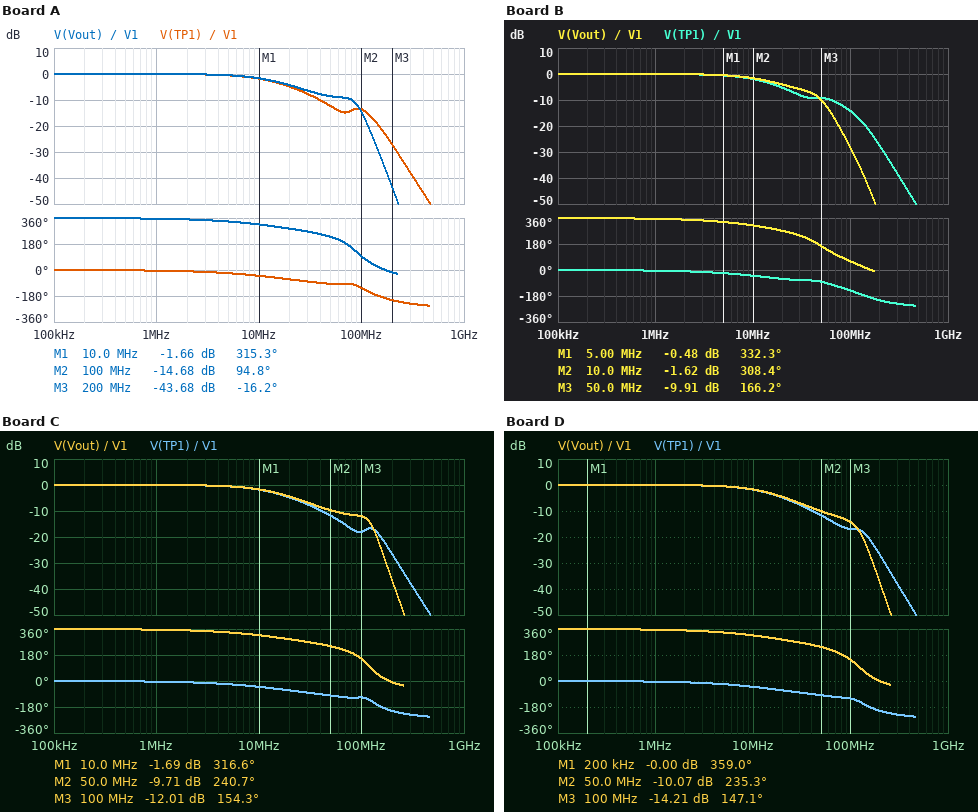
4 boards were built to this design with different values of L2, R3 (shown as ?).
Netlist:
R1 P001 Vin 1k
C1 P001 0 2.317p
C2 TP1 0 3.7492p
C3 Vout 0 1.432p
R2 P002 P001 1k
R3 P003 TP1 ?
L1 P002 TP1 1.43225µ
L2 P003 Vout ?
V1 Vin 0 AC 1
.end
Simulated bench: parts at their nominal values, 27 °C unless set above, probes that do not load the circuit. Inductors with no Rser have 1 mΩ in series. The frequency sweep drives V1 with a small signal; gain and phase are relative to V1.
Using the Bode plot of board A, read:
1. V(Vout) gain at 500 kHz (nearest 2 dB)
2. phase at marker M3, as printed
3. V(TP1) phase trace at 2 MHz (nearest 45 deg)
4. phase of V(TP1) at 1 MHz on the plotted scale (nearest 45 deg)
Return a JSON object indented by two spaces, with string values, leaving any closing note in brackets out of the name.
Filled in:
{
  "V(Vout) gain at 500 kHz": "0 dB",
  "phase at marker M3, as printed": "-16.2 deg",
  "V(TP1) phase trace at 2 MHz": "0 deg",
  "phase of V(TP1) at 1 MHz on the plotted scale": "0 deg"
}
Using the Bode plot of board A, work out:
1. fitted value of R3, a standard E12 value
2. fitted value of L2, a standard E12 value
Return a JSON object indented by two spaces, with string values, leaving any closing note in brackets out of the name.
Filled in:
{
  "fitted value of R3, a standard E12 value": "820 Ω",
  "fitted value of L2, a standard E12 value": "3.3 µH"
}
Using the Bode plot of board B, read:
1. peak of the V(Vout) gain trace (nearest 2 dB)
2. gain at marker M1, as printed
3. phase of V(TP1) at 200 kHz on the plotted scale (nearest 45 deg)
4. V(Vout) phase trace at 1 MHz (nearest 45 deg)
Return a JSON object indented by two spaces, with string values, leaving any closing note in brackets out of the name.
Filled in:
{
  "peak of the V(Vout) gain trace": "0 dB",
  "gain at marker M1, as printed": "-0.48 dB",
  "phase of V(TP1) at 200 kHz on the plotted scale": "0 deg",
  "V(Vout) phase trace at 1 MHz": "360 deg"
}
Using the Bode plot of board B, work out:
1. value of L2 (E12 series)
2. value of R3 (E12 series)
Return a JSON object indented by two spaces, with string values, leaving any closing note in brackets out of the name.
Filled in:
{
  "value of L2": "10 µH",
  "value of R3": "2.2 kΩ"
}
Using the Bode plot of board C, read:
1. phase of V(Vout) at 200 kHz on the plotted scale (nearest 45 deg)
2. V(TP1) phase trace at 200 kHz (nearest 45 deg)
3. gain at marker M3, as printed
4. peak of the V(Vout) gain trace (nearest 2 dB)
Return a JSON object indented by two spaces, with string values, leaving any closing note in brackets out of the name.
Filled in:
{
  "phase of V(Vout) at 200 kHz on the plotted scale": "360 deg",
  "V(TP1) phase trace at 200 kHz": "0 deg",
  "gain at marker M3, as printed": "-12.01 dB",
  "peak of the V(Vout) gain trace": "0 dB"
}
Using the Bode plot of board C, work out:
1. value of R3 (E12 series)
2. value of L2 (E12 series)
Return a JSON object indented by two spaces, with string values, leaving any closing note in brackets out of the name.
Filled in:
{
  "value of R3": "560 Ω",
  "value of L2": "1.8 µH"
}
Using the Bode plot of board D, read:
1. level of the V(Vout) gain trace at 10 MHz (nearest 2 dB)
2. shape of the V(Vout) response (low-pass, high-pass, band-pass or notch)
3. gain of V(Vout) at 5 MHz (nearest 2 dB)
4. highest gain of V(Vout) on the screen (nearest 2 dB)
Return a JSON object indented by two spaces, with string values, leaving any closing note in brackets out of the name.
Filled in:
{
  "level of the V(Vout) gain trace at 10 MHz": "-2 dB",
  "shape of the V(Vout) response": "low-pass",
  "gain of V(Vout) at 5 MHz": "0 dB",
  "highest gain of V(Vout) on the screen": "0 dB"
}
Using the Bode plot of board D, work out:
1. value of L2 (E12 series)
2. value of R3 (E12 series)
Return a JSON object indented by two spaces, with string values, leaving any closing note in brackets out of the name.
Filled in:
{
  "value of L2": "1.8 µH",
  "value of R3": "820 Ω"
}
